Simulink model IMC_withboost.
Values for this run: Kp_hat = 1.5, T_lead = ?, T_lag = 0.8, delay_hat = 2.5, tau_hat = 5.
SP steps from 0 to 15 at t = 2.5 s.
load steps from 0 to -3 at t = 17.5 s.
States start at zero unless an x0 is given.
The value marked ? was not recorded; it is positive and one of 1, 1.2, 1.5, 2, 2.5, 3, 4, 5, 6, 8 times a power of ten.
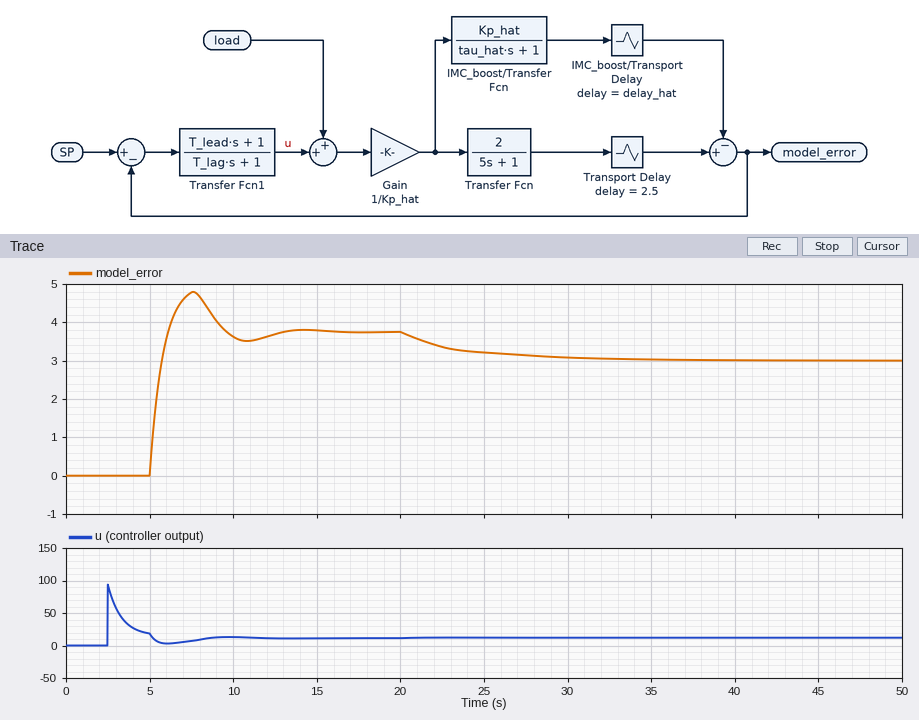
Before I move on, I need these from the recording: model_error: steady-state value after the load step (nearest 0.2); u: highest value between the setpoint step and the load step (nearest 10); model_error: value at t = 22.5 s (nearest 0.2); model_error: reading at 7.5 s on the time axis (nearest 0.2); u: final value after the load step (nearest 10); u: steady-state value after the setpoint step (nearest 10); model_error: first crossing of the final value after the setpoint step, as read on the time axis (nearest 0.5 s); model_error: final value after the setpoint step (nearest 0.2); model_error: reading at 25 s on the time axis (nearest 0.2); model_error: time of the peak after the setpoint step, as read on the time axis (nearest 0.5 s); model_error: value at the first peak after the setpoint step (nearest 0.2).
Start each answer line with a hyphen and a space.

- 3.0
- 90
- 3.4
- 4.8
- 10
- 10
- 6.0 s
- 3.8
- 3.2
- 7.5 s
- 4.8
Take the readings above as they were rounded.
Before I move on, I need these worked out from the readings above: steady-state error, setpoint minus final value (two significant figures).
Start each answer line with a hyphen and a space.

- 11
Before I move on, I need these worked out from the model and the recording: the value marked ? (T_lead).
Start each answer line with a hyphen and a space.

- 5
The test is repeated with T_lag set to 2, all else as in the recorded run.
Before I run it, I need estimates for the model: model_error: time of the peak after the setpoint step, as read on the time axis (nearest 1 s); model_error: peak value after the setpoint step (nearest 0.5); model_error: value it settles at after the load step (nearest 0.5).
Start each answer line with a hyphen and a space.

- 9 s
- 4.0
- 3.0
